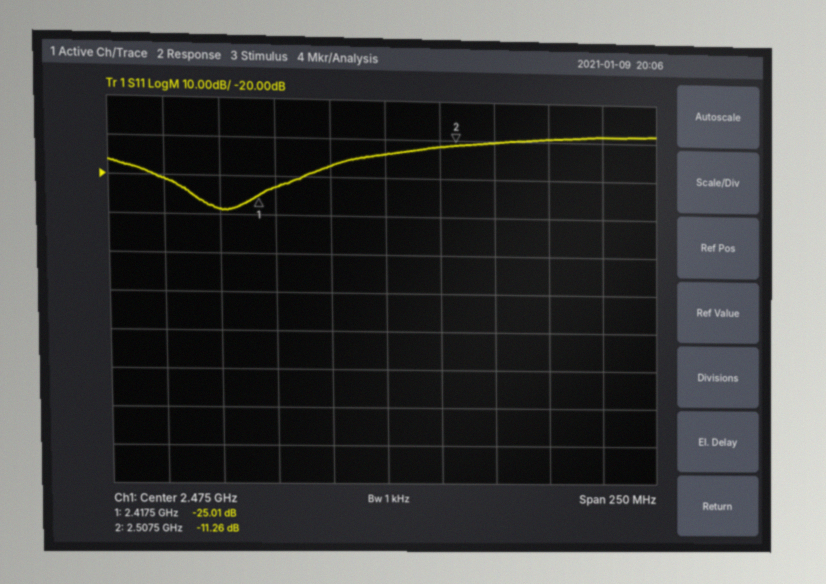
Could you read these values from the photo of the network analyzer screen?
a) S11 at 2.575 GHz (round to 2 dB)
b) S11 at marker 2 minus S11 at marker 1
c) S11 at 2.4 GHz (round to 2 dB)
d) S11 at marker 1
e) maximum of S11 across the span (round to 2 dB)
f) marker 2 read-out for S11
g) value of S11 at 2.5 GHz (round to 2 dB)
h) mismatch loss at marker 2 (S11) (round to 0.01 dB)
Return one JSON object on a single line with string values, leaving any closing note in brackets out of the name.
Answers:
{"S11 at 2.575 GHz": "-8 dB", "S11 at marker 2 minus S11 at marker 1": "13.75 dB", "S11 at 2.4 GHz": "-28 dB", "S11 at marker 1": "-25.01 dB", "maximum of S11 across the span": "-8 dB", "marker 2 read-out for S11": "-11.26 dB", "value of S11 at 2.5 GHz": "-12 dB", "mismatch loss at marker 2 (S11)": "0.34 dB"}
